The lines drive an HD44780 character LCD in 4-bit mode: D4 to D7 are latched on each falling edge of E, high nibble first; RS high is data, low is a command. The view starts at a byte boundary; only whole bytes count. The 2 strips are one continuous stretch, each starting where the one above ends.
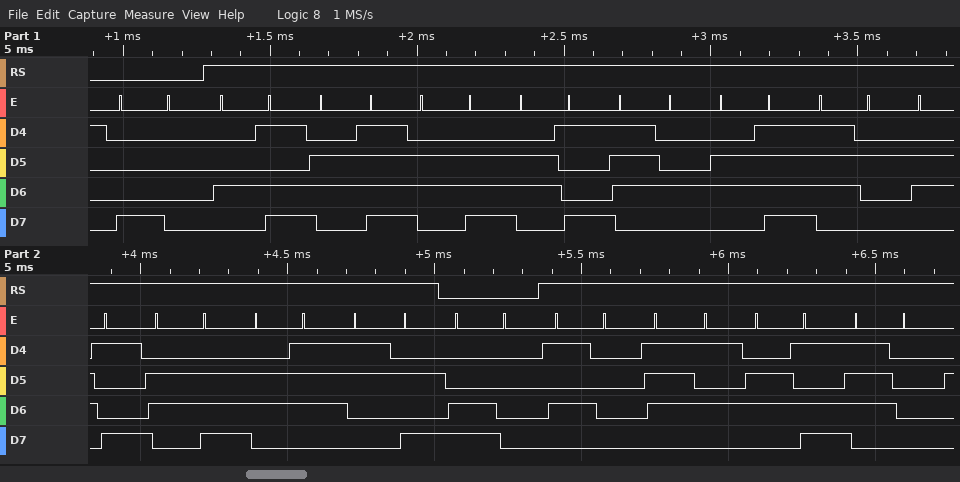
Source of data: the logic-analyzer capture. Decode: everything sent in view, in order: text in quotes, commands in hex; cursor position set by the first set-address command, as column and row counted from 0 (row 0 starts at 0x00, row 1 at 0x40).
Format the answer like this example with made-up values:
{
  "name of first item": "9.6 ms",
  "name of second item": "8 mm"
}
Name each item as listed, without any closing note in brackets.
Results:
{
  "everything sent in view, in order: text in quotes, commands in hex": "0x80 \"Monitoring:\" 0xC0 \"Pump\"",
  "cursor position set by the first set-address command, as column and row counted from 0": "column 0, row 0"
}
